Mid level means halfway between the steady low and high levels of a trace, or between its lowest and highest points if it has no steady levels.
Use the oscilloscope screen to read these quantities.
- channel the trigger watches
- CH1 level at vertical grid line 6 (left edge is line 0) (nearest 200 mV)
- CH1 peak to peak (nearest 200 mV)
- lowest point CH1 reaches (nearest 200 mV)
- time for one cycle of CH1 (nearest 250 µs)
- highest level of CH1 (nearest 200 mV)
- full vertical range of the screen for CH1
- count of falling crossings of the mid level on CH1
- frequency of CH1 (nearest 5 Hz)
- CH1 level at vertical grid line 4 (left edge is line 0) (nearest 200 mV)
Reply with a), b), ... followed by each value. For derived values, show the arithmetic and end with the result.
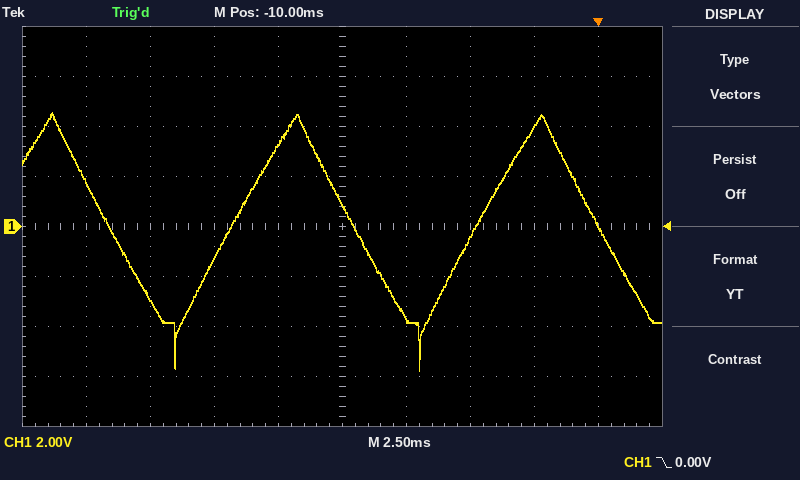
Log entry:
a) CH1
b) -3.6 V
c) 4.6 V − (-5.8 V) = 10.4 V
d) -5.8 V
e) 9.50 ms
f) 4.6 V
g) 16 V
h) 3
i) 1 / 9.50 ms ≈ 105 Hz
j) 3.2 V
